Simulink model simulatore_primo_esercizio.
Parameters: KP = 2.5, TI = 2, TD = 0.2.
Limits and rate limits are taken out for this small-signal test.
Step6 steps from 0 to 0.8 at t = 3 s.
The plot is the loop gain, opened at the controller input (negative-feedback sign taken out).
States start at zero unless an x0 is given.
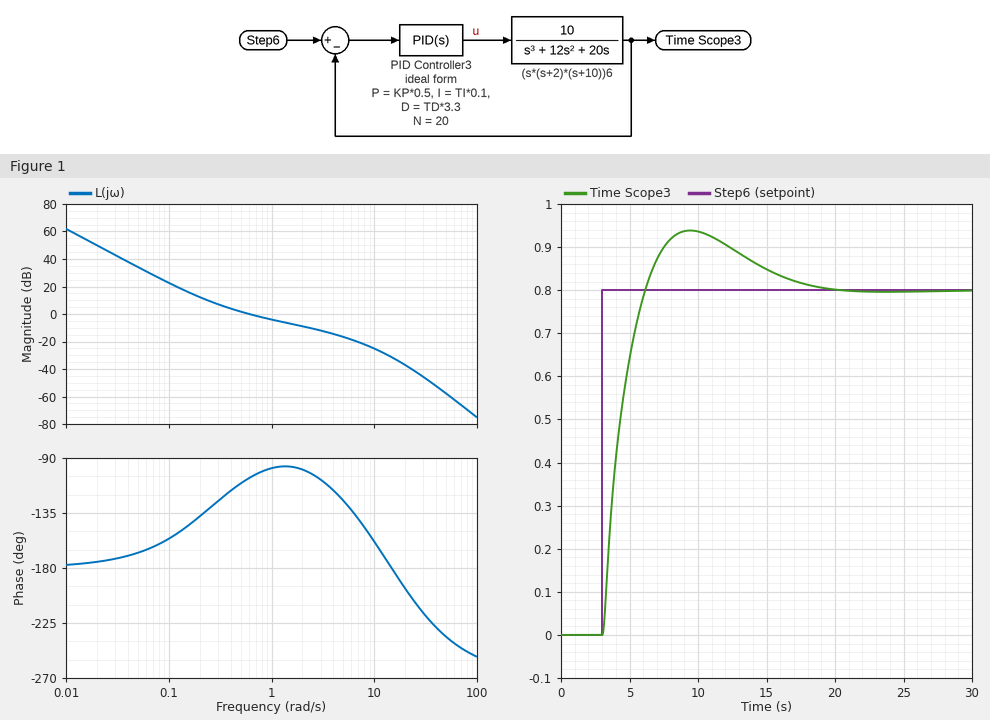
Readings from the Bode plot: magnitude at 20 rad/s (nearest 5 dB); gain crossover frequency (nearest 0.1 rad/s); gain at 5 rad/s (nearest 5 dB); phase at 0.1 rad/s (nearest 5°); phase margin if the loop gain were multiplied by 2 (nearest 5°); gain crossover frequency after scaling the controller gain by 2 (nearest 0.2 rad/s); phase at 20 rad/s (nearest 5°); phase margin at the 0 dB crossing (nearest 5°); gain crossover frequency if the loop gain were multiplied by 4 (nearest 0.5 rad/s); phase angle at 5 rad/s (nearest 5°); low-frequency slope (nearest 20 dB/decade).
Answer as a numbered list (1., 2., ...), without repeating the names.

1. -35 dB
2. 0.6 rad/s
3. -15 dB
4. -155°
5. 85°
6. 1.4 rad/s
7. -195°
8. 75°
9. 3.0 rad/s
10. -125°
11. -40 dB/decade
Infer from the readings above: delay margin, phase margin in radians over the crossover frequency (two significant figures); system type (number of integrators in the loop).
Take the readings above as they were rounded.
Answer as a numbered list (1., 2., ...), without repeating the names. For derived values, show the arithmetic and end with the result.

1. 75 × π / 180 / 0.6 = 2.2 s
2. 2
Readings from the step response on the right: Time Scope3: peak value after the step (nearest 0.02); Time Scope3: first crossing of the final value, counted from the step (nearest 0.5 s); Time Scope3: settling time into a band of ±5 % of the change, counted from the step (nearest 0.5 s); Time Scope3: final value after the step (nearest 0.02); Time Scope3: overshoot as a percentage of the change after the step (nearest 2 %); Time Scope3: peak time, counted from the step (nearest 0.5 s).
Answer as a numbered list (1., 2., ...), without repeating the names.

1. 0.94
2. 3.0 s
3. 12.5 s
4. 0.80
5. 18 %
6. 6.5 s
